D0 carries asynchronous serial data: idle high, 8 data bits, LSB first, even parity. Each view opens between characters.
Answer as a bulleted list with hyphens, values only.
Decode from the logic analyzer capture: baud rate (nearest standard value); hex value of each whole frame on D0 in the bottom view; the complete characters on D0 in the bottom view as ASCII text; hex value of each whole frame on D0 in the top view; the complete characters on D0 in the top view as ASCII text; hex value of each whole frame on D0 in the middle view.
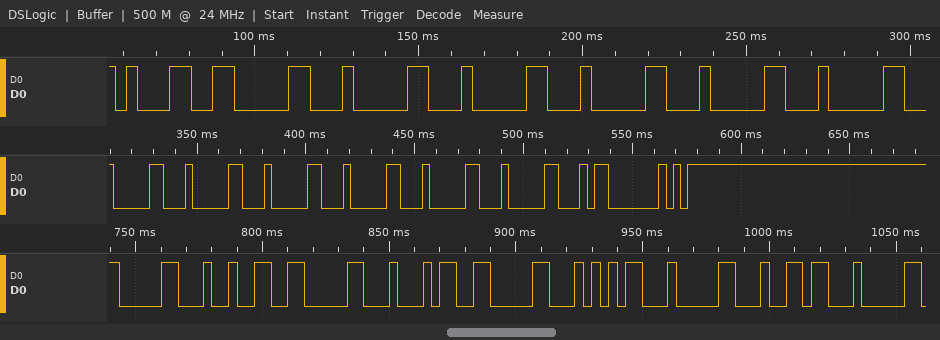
- 300 baud
- 30, 32, 30, 34, 30, 35, 30, 36
- "02040506"
- 31, 30, 30, 30, 30, 30
- "100000"
- 30, 30, 30, 30, 30, 30, 03, FD
